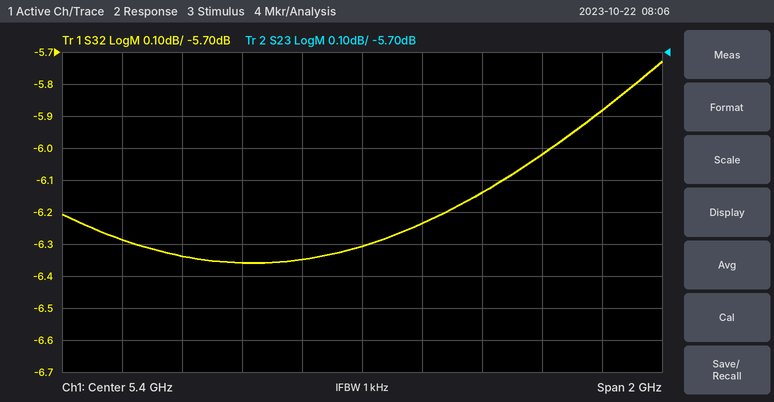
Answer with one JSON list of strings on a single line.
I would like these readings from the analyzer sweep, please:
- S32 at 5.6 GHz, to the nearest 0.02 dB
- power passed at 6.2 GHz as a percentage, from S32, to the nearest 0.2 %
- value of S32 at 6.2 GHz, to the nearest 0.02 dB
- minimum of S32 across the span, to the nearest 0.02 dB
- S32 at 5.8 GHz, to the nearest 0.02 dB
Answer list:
["-6.24 dB", "25.8 %", "-5.88 dB", "-6.36 dB", "-6.14 dB"]
